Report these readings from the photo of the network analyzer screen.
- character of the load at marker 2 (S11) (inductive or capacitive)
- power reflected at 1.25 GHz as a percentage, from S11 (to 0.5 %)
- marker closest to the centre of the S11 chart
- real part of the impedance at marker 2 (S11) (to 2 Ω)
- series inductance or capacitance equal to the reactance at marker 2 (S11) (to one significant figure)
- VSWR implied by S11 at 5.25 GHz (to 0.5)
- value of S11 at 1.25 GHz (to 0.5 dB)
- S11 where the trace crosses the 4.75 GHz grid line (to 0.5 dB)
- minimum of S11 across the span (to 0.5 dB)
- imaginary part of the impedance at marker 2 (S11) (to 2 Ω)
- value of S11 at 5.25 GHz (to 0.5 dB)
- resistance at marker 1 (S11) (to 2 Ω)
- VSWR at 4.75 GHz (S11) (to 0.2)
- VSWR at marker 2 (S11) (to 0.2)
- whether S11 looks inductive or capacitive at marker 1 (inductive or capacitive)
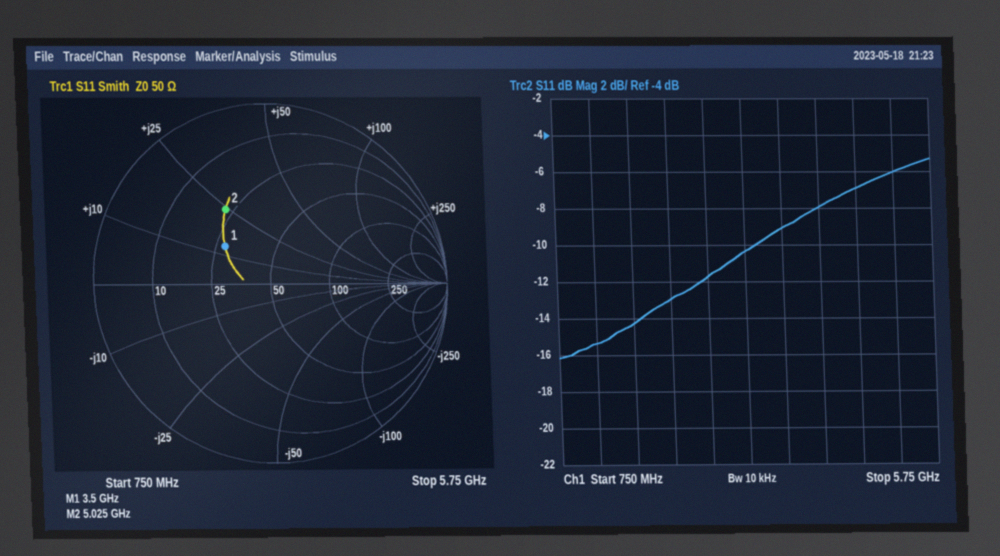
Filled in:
inductive
3.0 %
marker 1
22 Ω
800 pH
3.0
-15.5 dB
-7.0 dB
-16.0 dB
+24 Ω
-6.0 dB
28 Ω
2.6
2.8
inductive
